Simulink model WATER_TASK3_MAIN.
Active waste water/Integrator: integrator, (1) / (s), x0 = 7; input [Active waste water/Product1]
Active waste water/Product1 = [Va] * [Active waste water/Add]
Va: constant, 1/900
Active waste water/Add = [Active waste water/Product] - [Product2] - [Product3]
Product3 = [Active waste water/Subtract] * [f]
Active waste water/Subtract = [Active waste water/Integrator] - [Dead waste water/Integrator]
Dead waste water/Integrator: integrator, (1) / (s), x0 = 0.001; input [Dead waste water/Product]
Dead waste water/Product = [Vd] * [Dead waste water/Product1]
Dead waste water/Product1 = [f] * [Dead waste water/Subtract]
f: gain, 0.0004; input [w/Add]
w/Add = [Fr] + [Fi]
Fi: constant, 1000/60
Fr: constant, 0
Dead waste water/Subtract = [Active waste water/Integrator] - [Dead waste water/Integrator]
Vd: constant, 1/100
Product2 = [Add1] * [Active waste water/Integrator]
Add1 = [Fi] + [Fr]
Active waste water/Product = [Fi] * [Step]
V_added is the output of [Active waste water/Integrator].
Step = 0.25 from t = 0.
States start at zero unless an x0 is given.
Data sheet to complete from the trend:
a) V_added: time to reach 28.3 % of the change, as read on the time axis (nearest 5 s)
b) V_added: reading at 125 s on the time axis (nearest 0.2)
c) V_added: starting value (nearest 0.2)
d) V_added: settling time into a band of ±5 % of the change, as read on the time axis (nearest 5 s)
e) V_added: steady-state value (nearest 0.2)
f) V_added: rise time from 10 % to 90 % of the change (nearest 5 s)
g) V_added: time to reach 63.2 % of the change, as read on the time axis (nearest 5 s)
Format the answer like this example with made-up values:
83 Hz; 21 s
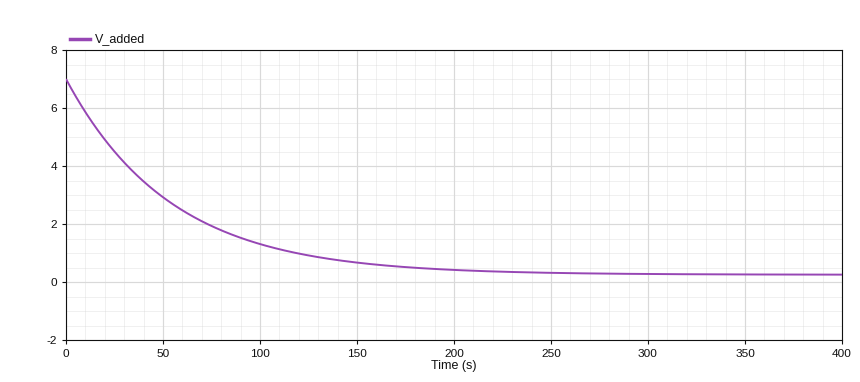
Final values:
20 s; 1.0; 7.0; 160 s; 0.2; 120 s; 55 s
